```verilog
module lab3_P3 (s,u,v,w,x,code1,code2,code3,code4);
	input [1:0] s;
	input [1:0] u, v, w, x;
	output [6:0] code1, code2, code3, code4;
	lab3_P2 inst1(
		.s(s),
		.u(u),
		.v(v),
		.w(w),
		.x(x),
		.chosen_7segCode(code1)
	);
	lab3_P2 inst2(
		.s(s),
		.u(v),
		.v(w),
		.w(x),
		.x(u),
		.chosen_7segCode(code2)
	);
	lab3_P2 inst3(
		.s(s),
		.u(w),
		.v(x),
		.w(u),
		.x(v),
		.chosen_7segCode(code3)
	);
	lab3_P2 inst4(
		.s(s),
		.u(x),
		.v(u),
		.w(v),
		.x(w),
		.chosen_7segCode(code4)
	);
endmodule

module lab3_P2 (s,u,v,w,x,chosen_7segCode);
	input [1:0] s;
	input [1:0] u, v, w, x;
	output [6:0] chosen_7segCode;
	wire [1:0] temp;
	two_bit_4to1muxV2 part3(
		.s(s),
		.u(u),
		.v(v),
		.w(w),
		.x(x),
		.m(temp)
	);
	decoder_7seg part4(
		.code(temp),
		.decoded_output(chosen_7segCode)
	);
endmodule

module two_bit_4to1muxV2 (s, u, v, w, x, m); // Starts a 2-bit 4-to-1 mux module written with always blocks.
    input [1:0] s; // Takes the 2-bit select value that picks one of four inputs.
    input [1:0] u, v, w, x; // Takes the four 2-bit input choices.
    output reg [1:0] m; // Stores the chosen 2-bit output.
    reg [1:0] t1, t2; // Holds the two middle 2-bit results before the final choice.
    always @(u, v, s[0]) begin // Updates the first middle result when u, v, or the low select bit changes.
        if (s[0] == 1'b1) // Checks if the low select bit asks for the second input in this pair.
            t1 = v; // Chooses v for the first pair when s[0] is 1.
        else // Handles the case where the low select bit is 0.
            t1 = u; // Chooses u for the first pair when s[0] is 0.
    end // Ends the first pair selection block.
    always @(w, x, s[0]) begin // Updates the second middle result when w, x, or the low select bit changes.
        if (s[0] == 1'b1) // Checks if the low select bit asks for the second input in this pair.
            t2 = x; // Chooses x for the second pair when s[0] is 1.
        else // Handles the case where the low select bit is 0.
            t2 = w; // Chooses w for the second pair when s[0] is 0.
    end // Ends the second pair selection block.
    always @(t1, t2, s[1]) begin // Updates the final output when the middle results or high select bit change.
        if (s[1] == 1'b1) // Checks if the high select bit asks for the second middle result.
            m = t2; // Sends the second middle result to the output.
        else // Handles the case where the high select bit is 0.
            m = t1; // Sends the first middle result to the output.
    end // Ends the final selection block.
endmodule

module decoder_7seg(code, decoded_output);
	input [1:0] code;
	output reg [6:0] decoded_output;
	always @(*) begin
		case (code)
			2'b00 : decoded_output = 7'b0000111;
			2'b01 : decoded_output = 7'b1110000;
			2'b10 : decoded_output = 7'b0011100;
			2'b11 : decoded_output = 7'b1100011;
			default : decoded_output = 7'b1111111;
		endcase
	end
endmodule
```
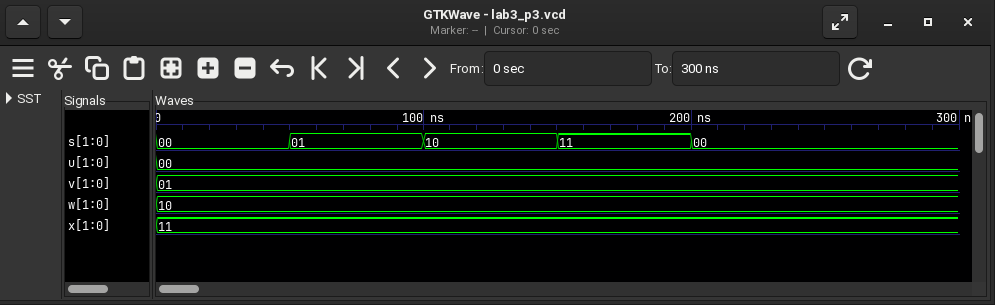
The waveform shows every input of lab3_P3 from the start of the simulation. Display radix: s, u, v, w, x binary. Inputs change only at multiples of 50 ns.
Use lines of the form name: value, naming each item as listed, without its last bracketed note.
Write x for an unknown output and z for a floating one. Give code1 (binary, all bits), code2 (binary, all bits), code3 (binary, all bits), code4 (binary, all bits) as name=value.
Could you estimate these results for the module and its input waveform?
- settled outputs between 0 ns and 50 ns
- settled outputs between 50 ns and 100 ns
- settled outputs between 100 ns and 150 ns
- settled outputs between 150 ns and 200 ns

settled outputs between 0 ns and 50 ns: code1=0000111, code2=1110000, code3=0011100, code4=1100011
settled outputs between 50 ns and 100 ns: code1=1110000, code2=0011100, code3=1100011, code4=0000111
settled outputs between 100 ns and 150 ns: code1=0011100, code2=1100011, code3=0000111, code4=1110000
settled outputs between 150 ns and 200 ns: code1=1100011, code2=0000111, code3=1110000, code4=0011100
